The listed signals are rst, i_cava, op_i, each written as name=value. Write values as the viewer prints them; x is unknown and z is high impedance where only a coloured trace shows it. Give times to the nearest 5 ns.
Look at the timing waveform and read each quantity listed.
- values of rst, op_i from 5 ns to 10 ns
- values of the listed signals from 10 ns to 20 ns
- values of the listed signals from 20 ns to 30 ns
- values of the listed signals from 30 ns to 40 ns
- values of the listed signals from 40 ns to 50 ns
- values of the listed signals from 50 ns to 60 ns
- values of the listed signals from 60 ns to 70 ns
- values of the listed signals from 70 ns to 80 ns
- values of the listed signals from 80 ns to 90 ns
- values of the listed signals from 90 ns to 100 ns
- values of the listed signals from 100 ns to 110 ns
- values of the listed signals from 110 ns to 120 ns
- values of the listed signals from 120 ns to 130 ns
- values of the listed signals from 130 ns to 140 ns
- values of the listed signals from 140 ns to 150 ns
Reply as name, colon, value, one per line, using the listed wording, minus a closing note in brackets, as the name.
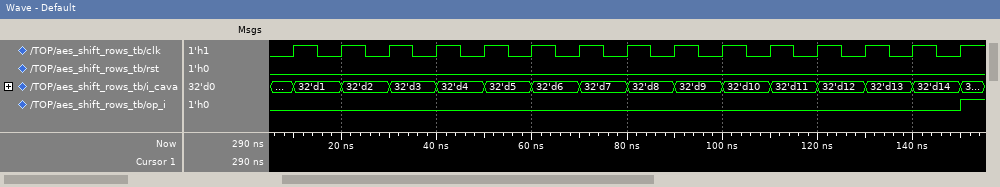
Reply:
values of rst, op_i from 5 ns to 10 ns: rst=0, op_i=0
values of the listed signals from 10 ns to 20 ns: rst=0, i_cava=32'd1, op_i=0
values of the listed signals from 20 ns to 30 ns: rst=0, i_cava=32'd2, op_i=0
values of the listed signals from 30 ns to 40 ns: rst=0, i_cava=32'd3, op_i=0
values of the listed signals from 40 ns to 50 ns: rst=0, i_cava=32'd4, op_i=0
values of the listed signals from 50 ns to 60 ns: rst=0, i_cava=32'd5, op_i=0
values of the listed signals from 60 ns to 70 ns: rst=0, i_cava=32'd6, op_i=0
values of the listed signals from 70 ns to 80 ns: rst=0, i_cava=32'd7, op_i=0
values of the listed signals from 80 ns to 90 ns: rst=0, i_cava=32'd8, op_i=0
values of the listed signals from 90 ns to 100 ns: rst=0, i_cava=32'd9, op_i=0
values of the listed signals from 100 ns to 110 ns: rst=0, i_cava=32'd10, op_i=0
values of the listed signals from 110 ns to 120 ns: rst=0, i_cava=32'd11, op_i=0
values of the listed signals from 120 ns to 130 ns: rst=0, i_cava=32'd12, op_i=0
values of the listed signals from 130 ns to 140 ns: rst=0, i_cava=32'd13, op_i=0
values of the listed signals from 140 ns to 150 ns: rst=0, i_cava=32'd14, op_i=0
